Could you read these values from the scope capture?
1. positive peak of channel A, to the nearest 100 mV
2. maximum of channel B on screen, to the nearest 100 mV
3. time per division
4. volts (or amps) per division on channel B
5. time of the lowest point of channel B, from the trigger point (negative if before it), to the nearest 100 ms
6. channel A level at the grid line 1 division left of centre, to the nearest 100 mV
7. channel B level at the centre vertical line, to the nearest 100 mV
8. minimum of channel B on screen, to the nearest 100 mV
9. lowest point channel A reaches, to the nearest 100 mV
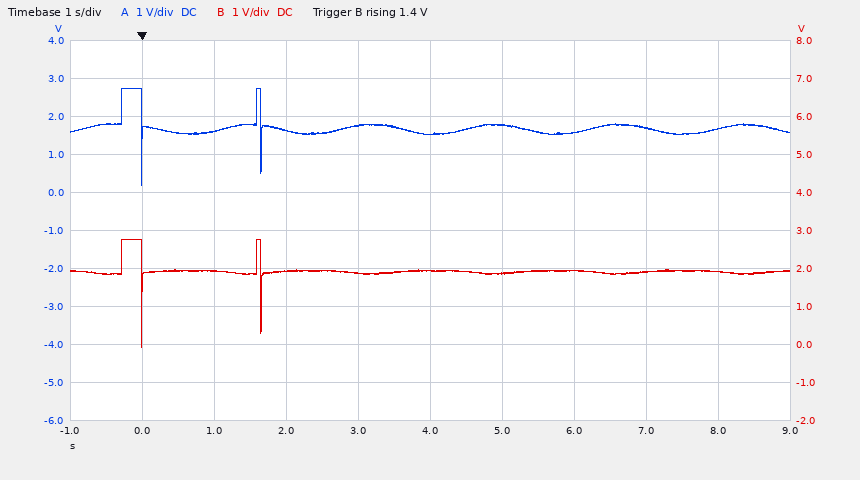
2.7 V
2.8 V
1 s
1 V
0.0 s
1.8 V
1.9 V
-100 mV
200 mV
